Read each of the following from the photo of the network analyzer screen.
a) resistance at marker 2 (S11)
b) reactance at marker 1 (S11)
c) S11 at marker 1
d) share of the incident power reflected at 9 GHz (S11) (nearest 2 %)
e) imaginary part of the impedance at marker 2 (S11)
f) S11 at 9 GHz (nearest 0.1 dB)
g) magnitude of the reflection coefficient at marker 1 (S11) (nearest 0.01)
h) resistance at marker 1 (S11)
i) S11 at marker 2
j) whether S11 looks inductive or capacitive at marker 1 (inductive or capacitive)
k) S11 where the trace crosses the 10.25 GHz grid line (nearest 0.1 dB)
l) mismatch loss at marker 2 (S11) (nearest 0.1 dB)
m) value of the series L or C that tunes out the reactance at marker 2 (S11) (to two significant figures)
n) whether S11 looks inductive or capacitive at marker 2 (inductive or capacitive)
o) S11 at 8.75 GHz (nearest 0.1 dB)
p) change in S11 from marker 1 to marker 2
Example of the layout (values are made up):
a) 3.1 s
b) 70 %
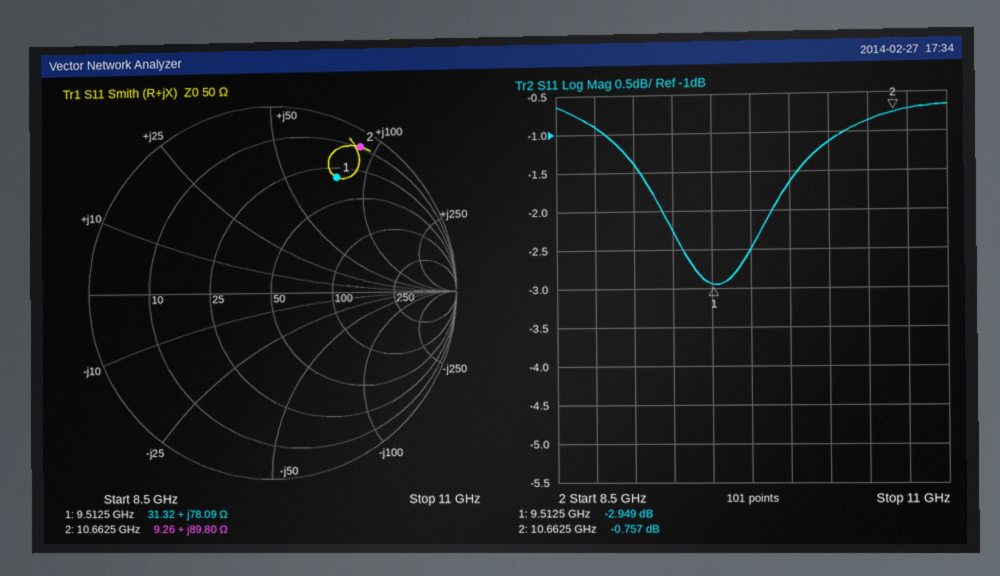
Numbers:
a) 9.26 Ω
b) +78.09 Ω
c) -2.949 dB
d) 72 %
e) +89.80 Ω
f) -1.4 dB
g) 0.71
h) 31.32 Ω
i) -0.757 dB
j) inductive
k) -1.1 dB
l) 8.0 dB
m) 170 fF
n) inductive
o) -0.9 dB
p) 2.192 dB
